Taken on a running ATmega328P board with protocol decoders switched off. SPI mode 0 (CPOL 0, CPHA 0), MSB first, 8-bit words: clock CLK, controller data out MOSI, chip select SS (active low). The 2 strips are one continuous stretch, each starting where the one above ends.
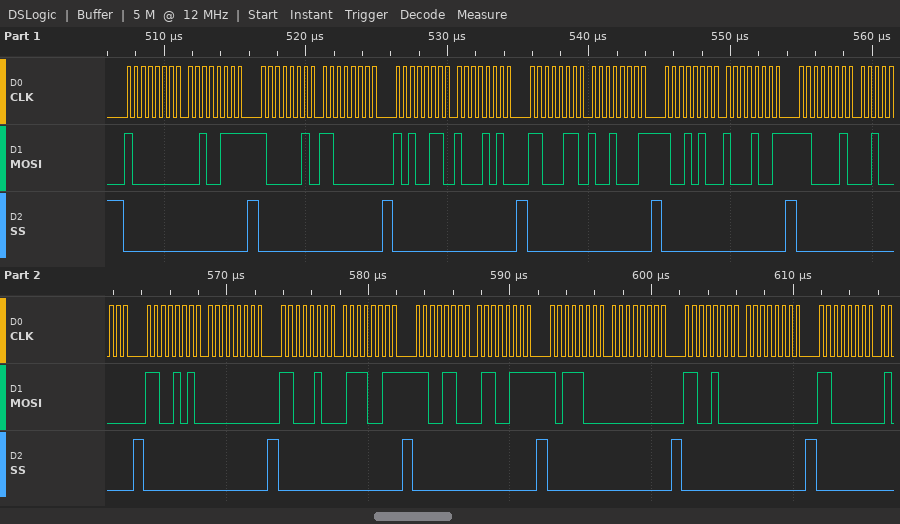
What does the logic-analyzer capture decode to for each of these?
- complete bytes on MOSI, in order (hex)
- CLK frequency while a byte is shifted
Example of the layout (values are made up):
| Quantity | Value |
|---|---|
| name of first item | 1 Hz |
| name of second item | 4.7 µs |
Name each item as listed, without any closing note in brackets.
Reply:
| Quantity | Value |
|---|---|
| complete bytes on MOSI, in order | 80 27 82 C0 A6 8A C6 91 94 89 C2 20 CA 00 C4 73 CC 67 B8 00 C8 00 C0 |
| CLK frequency while a byte is shifted | 2 MHz |
